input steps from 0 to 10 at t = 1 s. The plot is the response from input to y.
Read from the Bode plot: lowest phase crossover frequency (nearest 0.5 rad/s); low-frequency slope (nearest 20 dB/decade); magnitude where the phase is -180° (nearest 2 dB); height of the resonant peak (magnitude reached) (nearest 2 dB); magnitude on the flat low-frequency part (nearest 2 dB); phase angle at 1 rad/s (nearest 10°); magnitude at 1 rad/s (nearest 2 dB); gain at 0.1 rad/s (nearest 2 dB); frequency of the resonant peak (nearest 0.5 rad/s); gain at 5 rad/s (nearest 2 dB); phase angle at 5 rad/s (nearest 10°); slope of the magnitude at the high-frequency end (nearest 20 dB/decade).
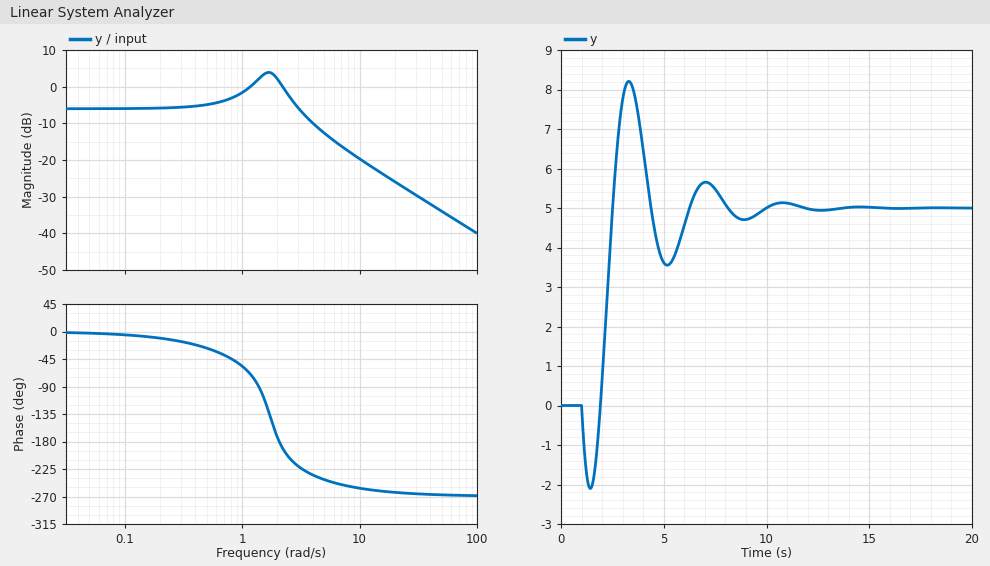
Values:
2.0 rad/s
0 dB/decade
2 dB
4 dB
-6 dB
-60°
-2 dB
-6 dB
1.5 rad/s
-12 dB
-240°
-20 dB/decade
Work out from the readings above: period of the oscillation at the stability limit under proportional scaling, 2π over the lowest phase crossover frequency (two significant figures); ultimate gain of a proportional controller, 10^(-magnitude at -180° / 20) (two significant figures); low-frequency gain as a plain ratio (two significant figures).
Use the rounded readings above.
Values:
3.1 s
0.79
0.50
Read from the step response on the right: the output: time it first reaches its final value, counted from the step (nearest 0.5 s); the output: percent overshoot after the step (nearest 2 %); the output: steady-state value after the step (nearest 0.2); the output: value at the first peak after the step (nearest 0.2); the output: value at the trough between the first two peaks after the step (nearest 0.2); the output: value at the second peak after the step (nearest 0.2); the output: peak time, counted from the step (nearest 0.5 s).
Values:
1.5 s
64 %
5.0
8.2
3.6
5.6
2.5 s
